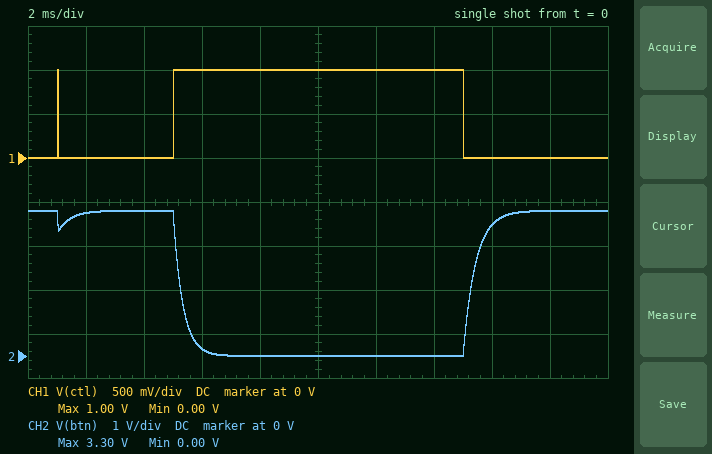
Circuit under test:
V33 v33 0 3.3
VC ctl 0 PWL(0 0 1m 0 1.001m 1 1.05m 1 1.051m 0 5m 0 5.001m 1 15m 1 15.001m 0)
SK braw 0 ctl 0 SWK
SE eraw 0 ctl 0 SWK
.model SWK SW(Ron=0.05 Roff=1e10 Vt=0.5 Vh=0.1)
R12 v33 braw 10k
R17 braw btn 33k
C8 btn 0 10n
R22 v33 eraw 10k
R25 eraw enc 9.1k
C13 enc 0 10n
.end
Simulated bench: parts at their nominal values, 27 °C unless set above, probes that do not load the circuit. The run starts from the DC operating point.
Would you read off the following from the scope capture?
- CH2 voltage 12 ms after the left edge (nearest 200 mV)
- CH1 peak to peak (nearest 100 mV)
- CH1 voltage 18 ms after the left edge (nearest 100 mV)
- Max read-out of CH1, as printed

0 V
1.0 V
0 V
1.00 V
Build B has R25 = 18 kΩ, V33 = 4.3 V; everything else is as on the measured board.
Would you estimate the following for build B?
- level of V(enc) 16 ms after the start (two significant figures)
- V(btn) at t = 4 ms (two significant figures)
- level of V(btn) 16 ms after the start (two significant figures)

4.2 V
4.3 V
3.9 V
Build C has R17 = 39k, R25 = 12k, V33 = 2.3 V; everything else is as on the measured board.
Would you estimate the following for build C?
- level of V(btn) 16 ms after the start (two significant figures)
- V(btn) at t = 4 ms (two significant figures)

2.0 V
2.3 V
